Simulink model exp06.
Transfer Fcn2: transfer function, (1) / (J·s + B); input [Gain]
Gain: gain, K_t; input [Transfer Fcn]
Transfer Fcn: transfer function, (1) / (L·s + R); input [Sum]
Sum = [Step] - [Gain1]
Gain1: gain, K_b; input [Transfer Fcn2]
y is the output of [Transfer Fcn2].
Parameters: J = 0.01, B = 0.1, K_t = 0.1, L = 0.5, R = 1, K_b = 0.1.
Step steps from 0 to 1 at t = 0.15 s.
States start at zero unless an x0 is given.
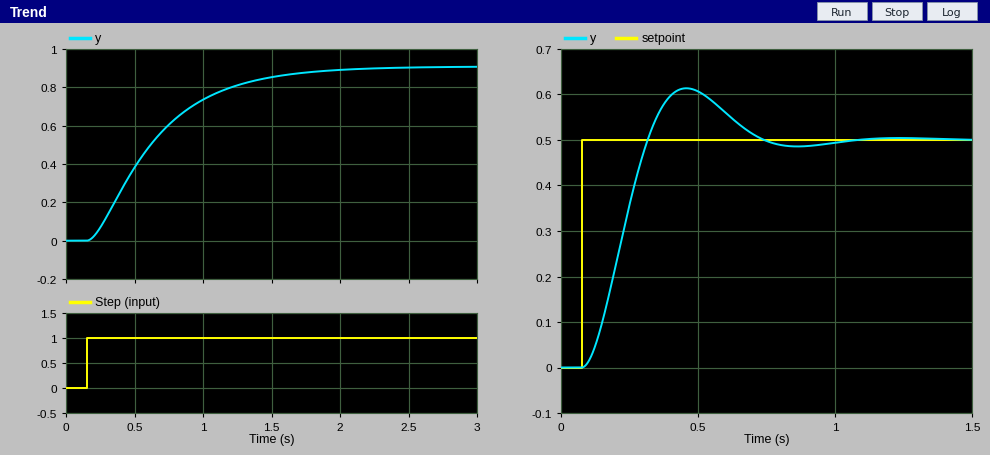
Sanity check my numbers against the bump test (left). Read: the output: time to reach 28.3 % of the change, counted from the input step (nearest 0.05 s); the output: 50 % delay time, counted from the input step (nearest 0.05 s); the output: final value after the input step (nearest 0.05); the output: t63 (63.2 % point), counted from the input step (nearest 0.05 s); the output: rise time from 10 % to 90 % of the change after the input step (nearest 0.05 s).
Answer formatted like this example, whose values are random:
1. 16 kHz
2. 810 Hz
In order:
1. 0.25 s
2. 0.40 s
3. 0.90
4. 0.55 s
5. 1.00 s
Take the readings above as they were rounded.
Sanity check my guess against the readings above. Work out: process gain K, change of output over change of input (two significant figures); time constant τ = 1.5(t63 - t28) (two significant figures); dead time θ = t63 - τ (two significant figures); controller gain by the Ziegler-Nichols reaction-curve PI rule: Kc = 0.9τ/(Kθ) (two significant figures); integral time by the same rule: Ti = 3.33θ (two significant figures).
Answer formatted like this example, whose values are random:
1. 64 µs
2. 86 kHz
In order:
1. 0.90
2. 0.45 s
3. 0.10 s
4. 4.5
5. 0.33 s
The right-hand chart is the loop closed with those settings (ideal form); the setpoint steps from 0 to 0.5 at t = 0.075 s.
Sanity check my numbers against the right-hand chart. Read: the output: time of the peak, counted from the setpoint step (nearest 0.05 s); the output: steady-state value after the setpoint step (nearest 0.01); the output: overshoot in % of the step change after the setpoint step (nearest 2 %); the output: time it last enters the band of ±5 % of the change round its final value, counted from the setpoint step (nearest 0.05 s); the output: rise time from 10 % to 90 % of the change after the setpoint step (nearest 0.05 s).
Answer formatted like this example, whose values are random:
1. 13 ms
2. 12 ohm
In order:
1. 0.40 s
2. 0.50
3. 22 %
4. 0.60 s
5. 0.15 s
